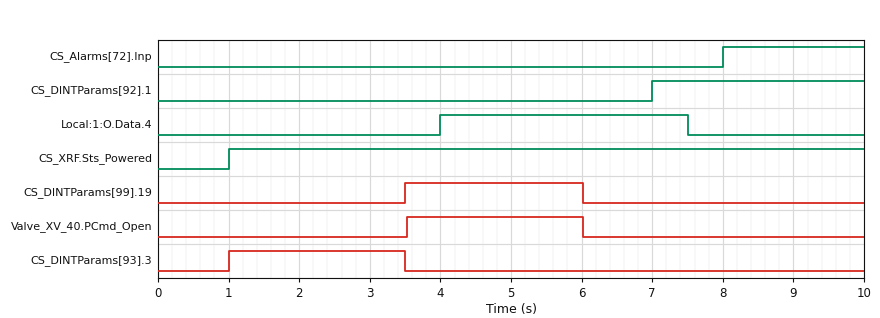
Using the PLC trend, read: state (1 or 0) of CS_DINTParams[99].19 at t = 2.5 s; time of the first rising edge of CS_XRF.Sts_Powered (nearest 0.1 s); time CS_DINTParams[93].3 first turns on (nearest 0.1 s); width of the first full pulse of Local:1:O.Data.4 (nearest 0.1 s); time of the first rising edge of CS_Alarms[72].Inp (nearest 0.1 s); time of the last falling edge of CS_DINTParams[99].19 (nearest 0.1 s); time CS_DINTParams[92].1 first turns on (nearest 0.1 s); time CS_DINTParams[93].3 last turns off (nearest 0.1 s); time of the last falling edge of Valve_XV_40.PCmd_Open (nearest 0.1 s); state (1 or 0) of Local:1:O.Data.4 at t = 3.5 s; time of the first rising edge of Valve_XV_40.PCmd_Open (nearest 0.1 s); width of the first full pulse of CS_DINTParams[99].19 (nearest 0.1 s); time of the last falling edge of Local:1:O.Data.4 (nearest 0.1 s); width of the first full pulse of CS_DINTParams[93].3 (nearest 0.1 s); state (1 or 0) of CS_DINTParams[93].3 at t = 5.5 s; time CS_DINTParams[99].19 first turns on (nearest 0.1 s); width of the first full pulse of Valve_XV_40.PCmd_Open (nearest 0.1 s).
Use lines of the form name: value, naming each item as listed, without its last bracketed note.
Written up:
state (1 or 0) of CS_DINTParams[99].19 at t = 2.5 s: 0
time of the first rising edge of CS_XRF.Sts_Powered: 1.0 s
time CS_DINTParams[93].3 first turns on: 1.0 s
width of the first full pulse of Local:1:O.Data.4: 3.5 s
time of the first rising edge of CS_Alarms[72].Inp: 8.0 s
time of the last falling edge of CS_DINTParams[99].19: 6.0 s
time CS_DINTParams[92].1 first turns on: 7.0 s
time CS_DINTParams[93].3 last turns off: 3.5 s
time of the last falling edge of Valve_XV_40.PCmd_Open: 6.0 s
state (1 or 0) of Local:1:O.Data.4 at t = 3.5 s: 0
time of the first rising edge of Valve_XV_40.PCmd_Open: 3.5 s
width of the first full pulse of CS_DINTParams[99].19: 2.5 s
time of the last falling edge of Local:1:O.Data.4: 7.5 s
width of the first full pulse of CS_DINTParams[93].3: 2.5 s
state (1 or 0) of CS_DINTParams[93].3 at t = 5.5 s: 0
time CS_DINTParams[99].19 first turns on: 3.5 s
width of the first full pulse of Valve_XV_40.PCmd_Open: 2.5 s
